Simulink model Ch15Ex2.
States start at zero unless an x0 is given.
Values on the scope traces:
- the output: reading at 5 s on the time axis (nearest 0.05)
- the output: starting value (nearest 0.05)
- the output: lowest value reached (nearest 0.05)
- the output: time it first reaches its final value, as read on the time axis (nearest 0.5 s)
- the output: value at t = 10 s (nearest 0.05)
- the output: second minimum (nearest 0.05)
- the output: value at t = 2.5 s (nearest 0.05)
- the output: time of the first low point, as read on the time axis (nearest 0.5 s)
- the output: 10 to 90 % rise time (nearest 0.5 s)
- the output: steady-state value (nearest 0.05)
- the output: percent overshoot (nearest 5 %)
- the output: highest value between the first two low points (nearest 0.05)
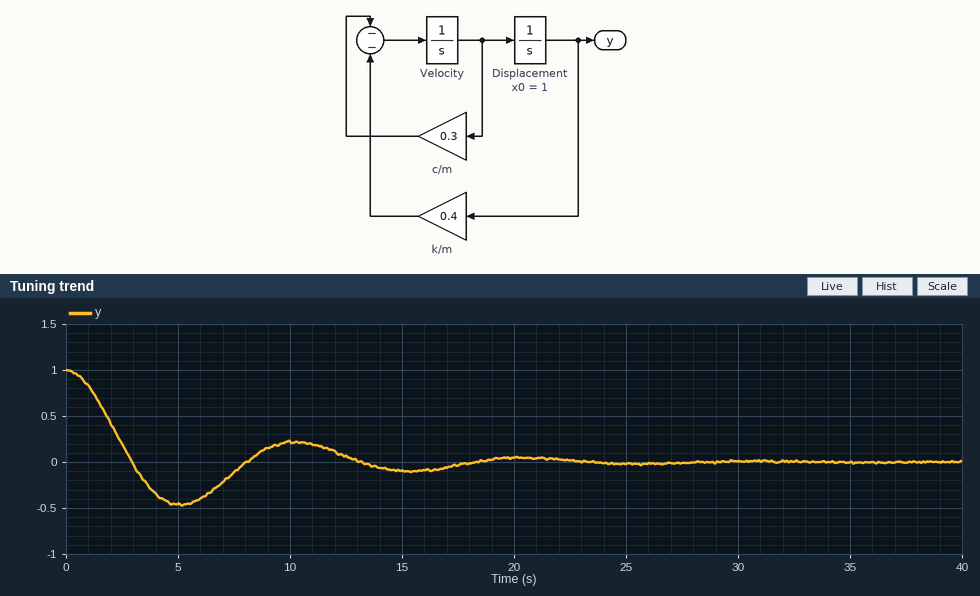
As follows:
-0.45
1.00
-0.45
3.0 s
0.20
-0.10
0.20
5.0 s
2.0 s
0.00
45 %
0.20
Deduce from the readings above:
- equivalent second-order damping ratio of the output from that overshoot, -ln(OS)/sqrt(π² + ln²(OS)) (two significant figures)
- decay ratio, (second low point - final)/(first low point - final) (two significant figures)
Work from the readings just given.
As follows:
0.25
0.22
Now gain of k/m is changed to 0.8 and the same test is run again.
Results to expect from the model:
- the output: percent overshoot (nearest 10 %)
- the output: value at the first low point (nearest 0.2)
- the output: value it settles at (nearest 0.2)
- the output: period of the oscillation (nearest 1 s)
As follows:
60 %
-0.6
0.0
7 s
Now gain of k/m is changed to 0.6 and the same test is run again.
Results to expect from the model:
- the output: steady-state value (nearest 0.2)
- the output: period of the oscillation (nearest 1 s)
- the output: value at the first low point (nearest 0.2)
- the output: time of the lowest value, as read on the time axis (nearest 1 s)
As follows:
0.0
8 s
-0.6
4 s
